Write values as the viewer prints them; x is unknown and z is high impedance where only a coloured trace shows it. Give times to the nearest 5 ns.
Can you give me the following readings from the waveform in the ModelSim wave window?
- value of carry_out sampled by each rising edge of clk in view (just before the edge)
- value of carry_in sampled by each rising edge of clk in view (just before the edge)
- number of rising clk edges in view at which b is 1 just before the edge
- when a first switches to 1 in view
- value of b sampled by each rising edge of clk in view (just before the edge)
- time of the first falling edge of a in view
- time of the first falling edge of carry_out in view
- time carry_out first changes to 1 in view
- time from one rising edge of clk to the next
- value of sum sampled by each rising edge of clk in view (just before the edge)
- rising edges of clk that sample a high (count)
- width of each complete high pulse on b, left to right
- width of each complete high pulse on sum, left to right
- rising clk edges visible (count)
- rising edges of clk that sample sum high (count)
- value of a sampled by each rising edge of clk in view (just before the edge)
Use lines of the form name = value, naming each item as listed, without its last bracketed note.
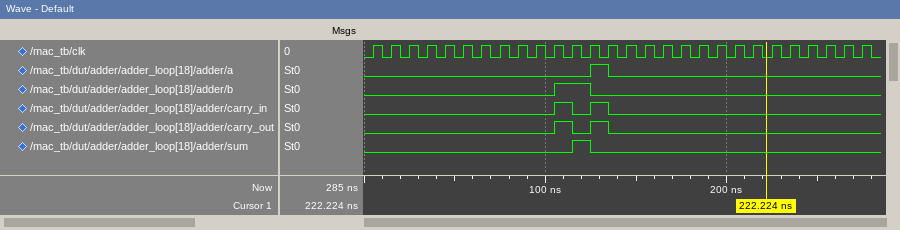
value of carry_out sampled by each rising edge of clk in view = 0 0 0 0 0 0 0 0 0 0 0 1 0 1 0 0 0 0 0 0 0 0 0 0 0 0 0 0
value of carry_in sampled by each rising edge of clk in view = 0 0 0 0 0 0 0 0 0 0 0 1 0 1 0 0 0 0 0 0 0 0 0 0 0 0 0 0
number of rising clk edges in view at which b is 1 just before the edge = 2
when a first switches to 1 in view = 125 ns
value of b sampled by each rising edge of clk in view = 0 0 0 0 0 0 0 0 0 0 0 1 1 0 0 0 0 0 0 0 0 0 0 0 0 0 0 0
time of the first falling edge of a in view = 135 ns
time of the first falling edge of carry_out in view = 115 ns
time carry_out first changes to 1 in view = 105 ns
time from one rising edge of clk to the next = 10 ns
value of sum sampled by each rising edge of clk in view = 0 0 0 0 0 0 0 0 0 0 0 0 1 0 0 0 0 0 0 0 0 0 0 0 0 0 0 0
rising edges of clk that sample a high = 1
width of each complete high pulse on b, left to right = 20 ns
width of each complete high pulse on sum, left to right = 10 ns
rising clk edges visible = 28
rising edges of clk that sample sum high = 1
value of a sampled by each rising edge of clk in view = 0 0 0 0 0 0 0 0 0 0 0 0 0 1 0 0 0 0 0 0 0 0 0 0 0 0 0 0
